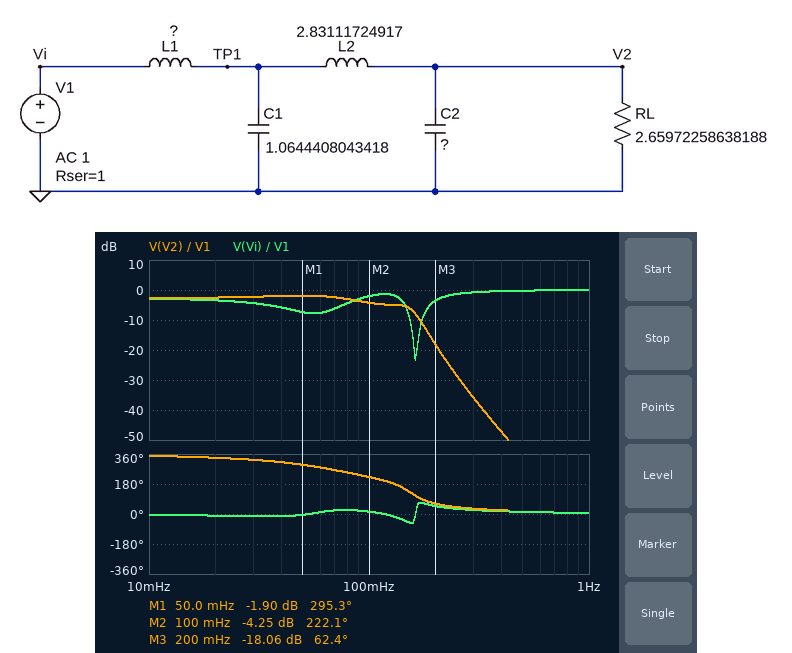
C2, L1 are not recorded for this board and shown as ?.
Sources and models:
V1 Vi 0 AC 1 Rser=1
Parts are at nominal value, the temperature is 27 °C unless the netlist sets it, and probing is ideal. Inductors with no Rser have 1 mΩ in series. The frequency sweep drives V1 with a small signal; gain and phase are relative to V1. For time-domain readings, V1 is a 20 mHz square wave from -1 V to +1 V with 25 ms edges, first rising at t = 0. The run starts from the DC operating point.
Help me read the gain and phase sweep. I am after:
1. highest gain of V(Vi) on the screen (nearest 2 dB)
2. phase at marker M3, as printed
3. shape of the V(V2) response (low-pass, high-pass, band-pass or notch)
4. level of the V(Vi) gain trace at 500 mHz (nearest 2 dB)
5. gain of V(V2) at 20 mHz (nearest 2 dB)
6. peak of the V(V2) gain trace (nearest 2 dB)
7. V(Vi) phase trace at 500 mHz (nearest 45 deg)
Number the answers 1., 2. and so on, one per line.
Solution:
1. 0 dB
2. 62.4 deg
3. low-pass
4. 0 dB
5. -2 dB
6. -2 dB
7. 0 deg
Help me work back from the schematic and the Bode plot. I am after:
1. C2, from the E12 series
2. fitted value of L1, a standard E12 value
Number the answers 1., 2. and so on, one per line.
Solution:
1. 1.5 F
2. 1.5 H
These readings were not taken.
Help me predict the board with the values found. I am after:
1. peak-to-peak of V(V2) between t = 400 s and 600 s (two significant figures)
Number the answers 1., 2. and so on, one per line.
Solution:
1. 1.9 V
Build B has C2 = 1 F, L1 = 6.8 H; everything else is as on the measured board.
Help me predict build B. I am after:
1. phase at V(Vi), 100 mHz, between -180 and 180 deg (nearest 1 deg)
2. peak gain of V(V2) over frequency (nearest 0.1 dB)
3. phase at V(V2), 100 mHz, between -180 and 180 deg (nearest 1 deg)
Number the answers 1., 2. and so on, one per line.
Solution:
1. 11 deg
2. -2.0 dB
3. -160 deg
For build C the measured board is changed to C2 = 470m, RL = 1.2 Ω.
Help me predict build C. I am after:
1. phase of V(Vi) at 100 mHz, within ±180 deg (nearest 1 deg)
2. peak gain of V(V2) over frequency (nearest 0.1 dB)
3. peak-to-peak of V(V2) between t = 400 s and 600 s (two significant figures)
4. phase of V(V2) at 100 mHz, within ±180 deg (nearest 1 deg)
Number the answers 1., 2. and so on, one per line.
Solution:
1. -3 deg
2. -5.3 dB
3. 1.3 V
4. -98 deg
